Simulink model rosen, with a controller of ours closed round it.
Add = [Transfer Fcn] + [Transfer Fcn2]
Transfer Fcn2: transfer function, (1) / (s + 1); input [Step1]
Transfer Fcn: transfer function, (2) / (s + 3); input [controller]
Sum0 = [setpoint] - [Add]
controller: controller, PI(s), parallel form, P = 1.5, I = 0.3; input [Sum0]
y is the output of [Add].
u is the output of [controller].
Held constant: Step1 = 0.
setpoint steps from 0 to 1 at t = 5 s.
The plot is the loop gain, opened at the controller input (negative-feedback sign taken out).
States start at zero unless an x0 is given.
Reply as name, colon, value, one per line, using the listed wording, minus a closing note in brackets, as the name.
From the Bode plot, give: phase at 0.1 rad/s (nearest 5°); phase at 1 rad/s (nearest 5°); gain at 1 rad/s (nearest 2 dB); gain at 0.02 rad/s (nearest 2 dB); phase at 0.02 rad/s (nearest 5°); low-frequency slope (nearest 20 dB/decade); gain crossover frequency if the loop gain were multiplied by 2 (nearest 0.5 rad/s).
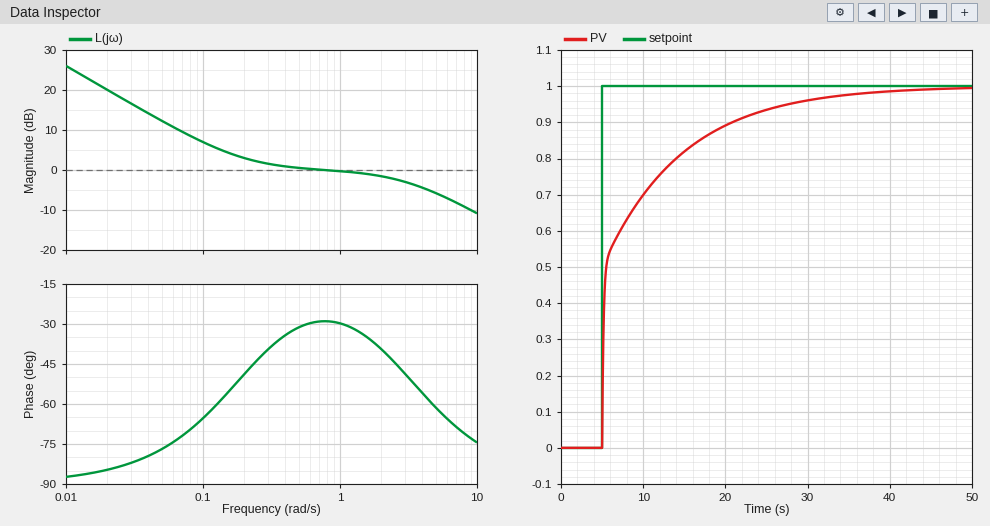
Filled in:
phase at 0.1 rad/s: -65°
phase at 1 rad/s: -30°
gain at 1 rad/s: 0 dB
gain at 0.02 rad/s: 20 dB
phase at 0.02 rad/s: -85°
low-frequency slope: -20 dB/decade
gain crossover frequency if the loop gain were multiplied by 2: 5.0 rad/s
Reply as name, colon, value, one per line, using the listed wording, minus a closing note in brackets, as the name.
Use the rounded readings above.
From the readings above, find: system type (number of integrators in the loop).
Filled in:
system type: 1
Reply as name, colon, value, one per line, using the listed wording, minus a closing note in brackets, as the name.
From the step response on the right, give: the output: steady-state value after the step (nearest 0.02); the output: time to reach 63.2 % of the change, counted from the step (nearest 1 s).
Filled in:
the output: steady-state value after the step: 1.00
the output: time to reach 63.2 % of the change, counted from the step: 3 s
